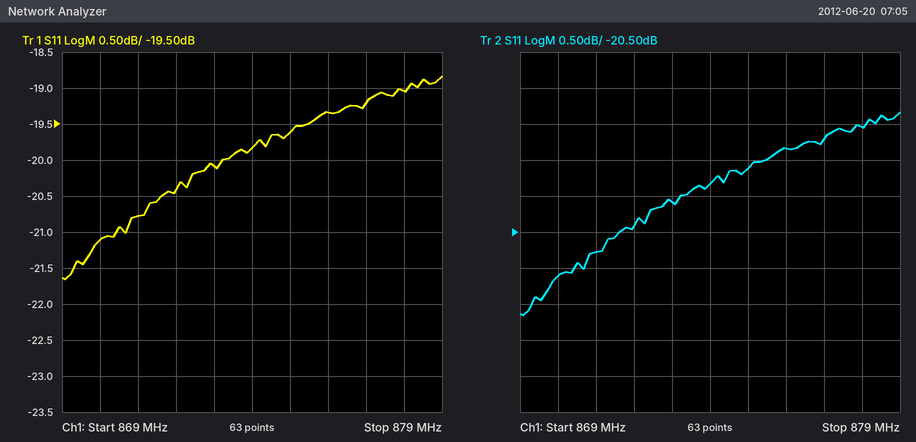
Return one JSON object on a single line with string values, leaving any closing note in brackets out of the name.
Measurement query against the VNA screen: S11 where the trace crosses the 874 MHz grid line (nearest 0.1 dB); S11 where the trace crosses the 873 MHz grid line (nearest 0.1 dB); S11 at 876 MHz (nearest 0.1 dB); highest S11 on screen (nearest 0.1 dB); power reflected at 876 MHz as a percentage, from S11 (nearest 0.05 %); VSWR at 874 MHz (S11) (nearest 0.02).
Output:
{"S11 where the trace crosses the 874 MHz grid line": "-19.8 dB", "S11 where the trace crosses the 873 MHz grid line": "-20.1 dB", "S11 at 876 MHz": "-19.3 dB", "highest S11 on screen": "-18.8 dB", "power reflected at 876 MHz as a percentage, from S11": "1.15 %", "VSWR at 874 MHz (S11)": "1.22"}
